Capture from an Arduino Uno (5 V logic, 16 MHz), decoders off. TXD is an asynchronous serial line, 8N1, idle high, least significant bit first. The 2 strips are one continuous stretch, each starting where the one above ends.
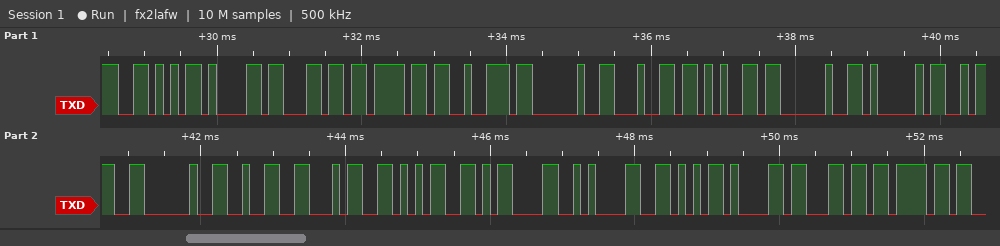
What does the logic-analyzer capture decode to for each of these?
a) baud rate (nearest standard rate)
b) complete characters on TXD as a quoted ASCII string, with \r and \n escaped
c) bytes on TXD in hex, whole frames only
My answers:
9600 baud
"Valor de A: 245\r\nValo"
56 61 6C 6F 72 20 64 65 20 41 3A 20 32 34 35 0D 0A 56 61 6C 6F
